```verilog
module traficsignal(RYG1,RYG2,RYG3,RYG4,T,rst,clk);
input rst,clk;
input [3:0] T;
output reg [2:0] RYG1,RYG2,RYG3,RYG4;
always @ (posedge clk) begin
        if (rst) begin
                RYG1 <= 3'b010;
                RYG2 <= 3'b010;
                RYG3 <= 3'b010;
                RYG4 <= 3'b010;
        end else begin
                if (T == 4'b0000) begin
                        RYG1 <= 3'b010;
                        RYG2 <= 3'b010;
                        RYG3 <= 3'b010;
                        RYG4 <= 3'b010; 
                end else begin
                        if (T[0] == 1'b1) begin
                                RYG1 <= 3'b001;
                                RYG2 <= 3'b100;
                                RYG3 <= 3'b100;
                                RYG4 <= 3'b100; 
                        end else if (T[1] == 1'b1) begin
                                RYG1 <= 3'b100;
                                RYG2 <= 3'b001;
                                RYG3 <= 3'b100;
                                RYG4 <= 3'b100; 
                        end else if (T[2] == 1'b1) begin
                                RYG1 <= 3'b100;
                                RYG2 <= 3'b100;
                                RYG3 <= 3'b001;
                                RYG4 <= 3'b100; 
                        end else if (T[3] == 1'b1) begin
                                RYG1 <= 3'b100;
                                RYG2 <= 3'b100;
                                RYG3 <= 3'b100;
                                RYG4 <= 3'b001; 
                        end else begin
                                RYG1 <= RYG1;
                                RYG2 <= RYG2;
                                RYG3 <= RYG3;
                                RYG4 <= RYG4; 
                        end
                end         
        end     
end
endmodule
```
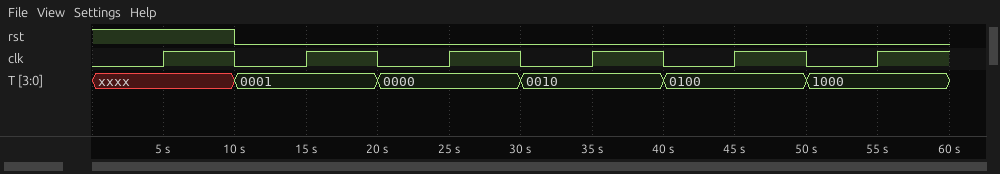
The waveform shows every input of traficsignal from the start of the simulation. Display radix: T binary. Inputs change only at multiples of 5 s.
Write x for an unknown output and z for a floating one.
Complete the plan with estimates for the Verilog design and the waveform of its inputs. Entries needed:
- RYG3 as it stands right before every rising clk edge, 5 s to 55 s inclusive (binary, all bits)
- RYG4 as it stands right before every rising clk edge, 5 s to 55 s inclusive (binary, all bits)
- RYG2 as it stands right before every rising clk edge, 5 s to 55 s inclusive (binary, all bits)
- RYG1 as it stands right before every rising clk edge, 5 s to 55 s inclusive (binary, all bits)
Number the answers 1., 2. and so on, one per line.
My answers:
1. x, 010, 100, 010, 100, 001
2. x, 010, 100, 010, 100, 100
3. x, 010, 100, 010, 001, 100
4. x, 010, 001, 010, 100, 100
